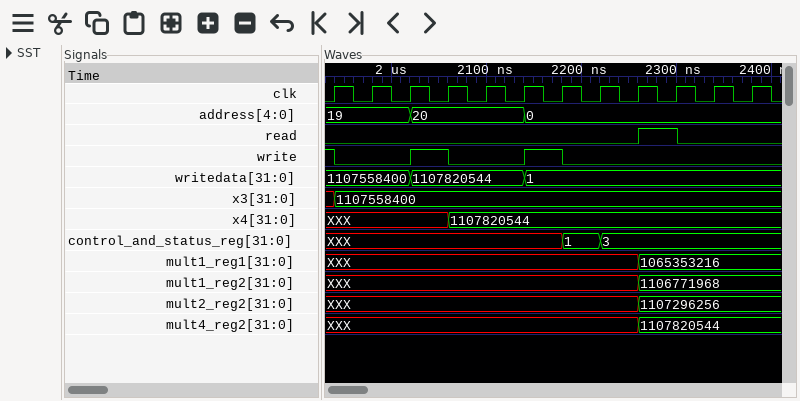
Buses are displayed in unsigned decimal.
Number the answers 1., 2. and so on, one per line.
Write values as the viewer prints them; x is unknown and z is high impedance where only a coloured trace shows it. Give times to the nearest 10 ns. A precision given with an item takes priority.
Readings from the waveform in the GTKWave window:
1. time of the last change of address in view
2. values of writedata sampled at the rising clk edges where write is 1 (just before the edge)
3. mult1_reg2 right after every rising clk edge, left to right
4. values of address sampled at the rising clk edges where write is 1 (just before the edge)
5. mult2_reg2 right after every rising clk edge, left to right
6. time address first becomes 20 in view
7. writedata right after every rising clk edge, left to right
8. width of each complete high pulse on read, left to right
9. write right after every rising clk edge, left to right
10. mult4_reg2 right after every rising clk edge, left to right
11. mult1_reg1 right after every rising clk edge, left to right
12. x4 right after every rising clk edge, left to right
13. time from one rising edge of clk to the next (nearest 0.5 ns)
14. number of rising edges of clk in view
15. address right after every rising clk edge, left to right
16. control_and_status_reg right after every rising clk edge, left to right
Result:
1. 2140 ns
2. 1107558400, 1107820544, 1
3. XXX, XXX, XXX, XXX, XXX, XXX, XXX, XXX, 1106771968, 1106771968, 1106771968, 1106771968
4. 19, 20, 0
5. XXX, XXX, XXX, XXX, XXX, XXX, XXX, XXX, 1107296256, 1107296256, 1107296256, 1107296256
6. 2020 ns
7. 1107558400, 1107558400, 1107820544, 1107820544, 1107820544, 1, 1, 1, 1, 1, 1, 1
8. 40 ns
9. 0 0 1 0 0 1 0 0 0 0 0 0
10. XXX, XXX, XXX, XXX, XXX, XXX, XXX, XXX, 1107820544, 1107820544, 1107820544, 1107820544
11. XXX, XXX, XXX, XXX, XXX, XXX, XXX, XXX, 1065353216, 1065353216, 1065353216, 1065353216
12. XXX, XXX, XXX, 1107820544, 1107820544, 1107820544, 1107820544, 1107820544, 1107820544, 1107820544, 1107820544, 1107820544
13. 40 ns
14. 12
15. 19, 19, 20, 20, 20, 0, 0, 0, 0, 0, 0, 0
16. XXX, XXX, XXX, XXX, XXX, XXX, 1, 3, 3, 3, 3, 3
